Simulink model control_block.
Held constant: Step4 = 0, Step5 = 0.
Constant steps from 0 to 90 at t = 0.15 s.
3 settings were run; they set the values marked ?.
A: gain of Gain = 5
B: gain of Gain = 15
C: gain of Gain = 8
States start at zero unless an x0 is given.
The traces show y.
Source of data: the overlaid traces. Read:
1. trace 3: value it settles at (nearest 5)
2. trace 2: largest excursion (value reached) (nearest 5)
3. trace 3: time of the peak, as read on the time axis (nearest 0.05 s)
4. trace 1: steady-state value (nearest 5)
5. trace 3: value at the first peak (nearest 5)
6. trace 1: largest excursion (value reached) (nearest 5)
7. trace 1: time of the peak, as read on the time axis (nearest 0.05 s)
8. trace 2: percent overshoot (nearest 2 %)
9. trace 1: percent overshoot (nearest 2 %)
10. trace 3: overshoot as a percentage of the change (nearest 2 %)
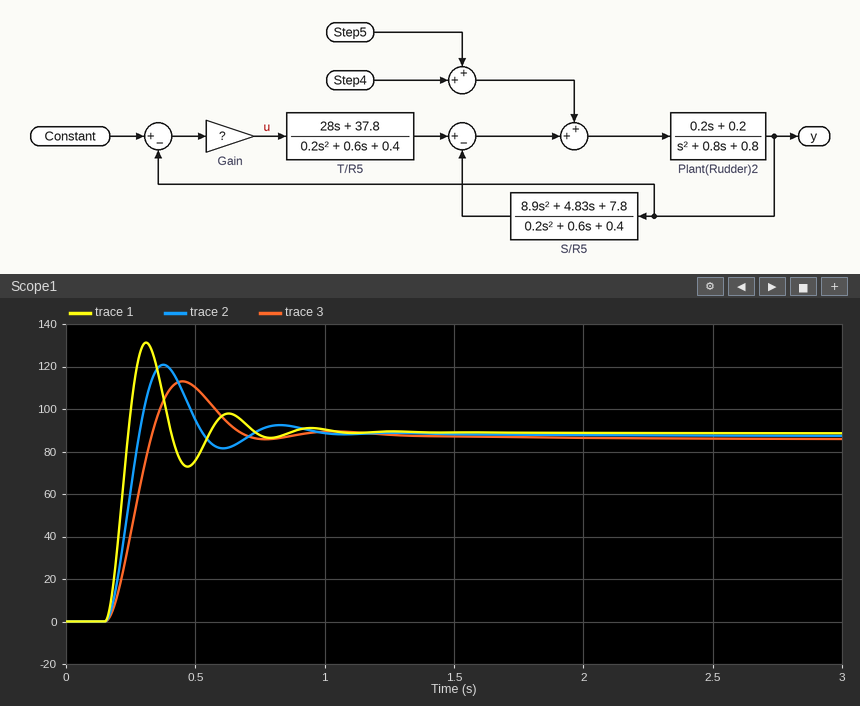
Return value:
85
120
0.45 s
90
115
130
0.30 s
38 %
48 %
32 %
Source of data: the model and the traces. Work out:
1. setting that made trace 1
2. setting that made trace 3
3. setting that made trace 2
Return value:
B
A
C
